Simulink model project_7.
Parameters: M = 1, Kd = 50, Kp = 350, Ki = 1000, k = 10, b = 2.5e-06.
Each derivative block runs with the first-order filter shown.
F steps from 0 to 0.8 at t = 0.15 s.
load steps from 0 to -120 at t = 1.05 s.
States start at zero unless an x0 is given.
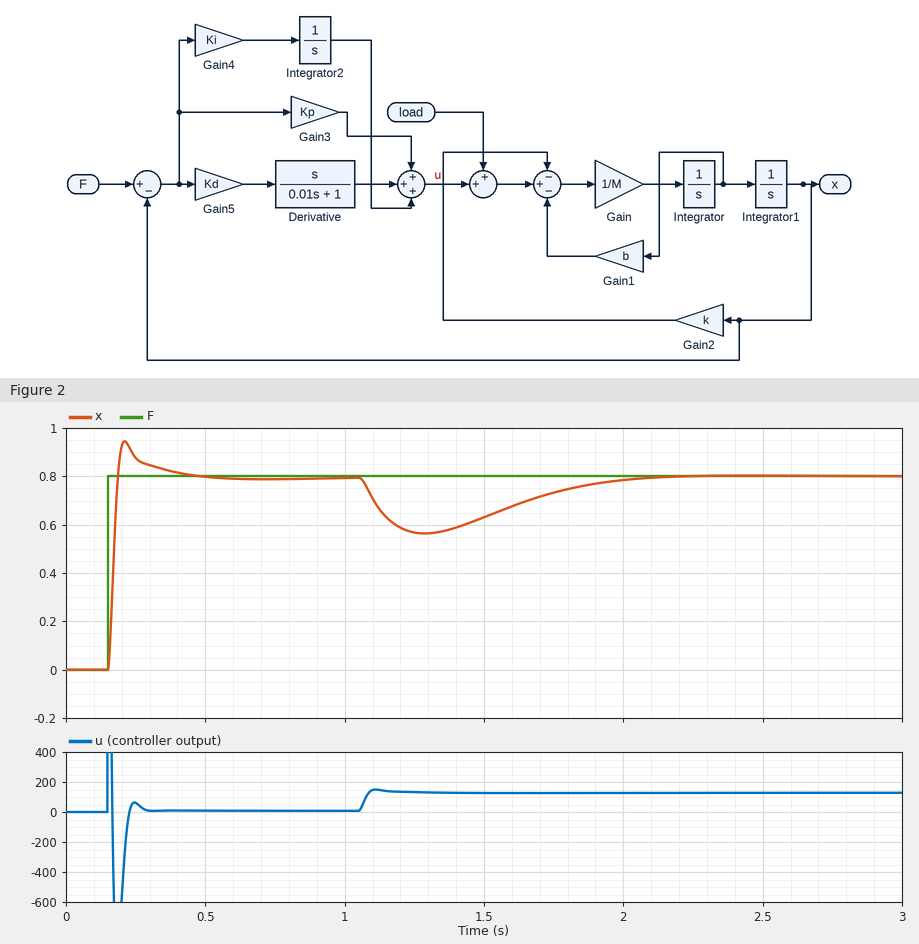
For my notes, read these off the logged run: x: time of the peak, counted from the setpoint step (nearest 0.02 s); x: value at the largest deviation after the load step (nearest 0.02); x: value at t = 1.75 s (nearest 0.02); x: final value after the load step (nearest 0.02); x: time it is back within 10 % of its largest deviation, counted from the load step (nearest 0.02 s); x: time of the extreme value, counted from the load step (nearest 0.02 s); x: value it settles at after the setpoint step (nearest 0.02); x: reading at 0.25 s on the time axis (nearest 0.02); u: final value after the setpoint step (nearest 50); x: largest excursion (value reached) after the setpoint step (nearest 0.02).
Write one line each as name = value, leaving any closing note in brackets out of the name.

x: time of the peak, counted from the setpoint step = 0.06 s
x: value at the largest deviation after the load step = 0.56
x: value at t = 1.75 s = 0.74
x: final value after the load step = 0.80
x: time it is back within 10 % of its largest deviation, counted from the load step = 0.90 s
x: time of the extreme value, counted from the load step = 0.24 s
x: value it settles at after the setpoint step = 0.80
x: reading at 0.25 s on the time axis = 0.88
u: final value after the setpoint step = 0
x: largest excursion (value reached) after the setpoint step = 0.94
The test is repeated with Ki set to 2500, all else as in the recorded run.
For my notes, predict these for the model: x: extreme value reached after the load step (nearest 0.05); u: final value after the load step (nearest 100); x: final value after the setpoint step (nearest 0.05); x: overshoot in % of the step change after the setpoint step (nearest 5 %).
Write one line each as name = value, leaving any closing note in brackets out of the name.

x: extreme value reached after the load step = 0.60
u: final value after the load step = 100
x: final value after the setpoint step = 0.80
x: overshoot in % of the step change after the setpoint step = 20 %
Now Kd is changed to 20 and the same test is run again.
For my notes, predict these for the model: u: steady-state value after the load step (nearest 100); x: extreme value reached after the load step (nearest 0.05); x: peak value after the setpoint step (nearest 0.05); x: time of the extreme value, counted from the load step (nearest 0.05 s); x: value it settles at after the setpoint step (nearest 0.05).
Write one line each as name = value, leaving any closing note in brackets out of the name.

u: steady-state value after the load step = 100
x: extreme value reached after the load step = 0.45
x: peak value after the setpoint step = 1.10
x: time of the extreme value, counted from the load step = 0.15 s
x: value it settles at after the setpoint step = 0.80
